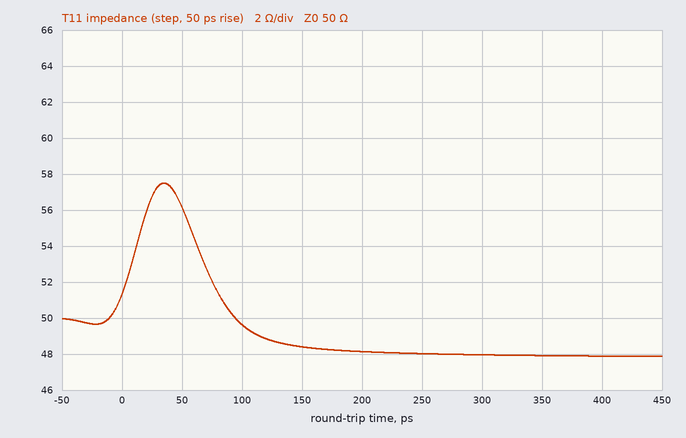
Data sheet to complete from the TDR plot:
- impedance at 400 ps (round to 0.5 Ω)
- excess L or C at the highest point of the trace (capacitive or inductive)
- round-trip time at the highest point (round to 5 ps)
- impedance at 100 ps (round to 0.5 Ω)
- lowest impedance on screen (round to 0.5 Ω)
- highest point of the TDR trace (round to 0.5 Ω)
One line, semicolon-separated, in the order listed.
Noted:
48.0 Ω; inductive; 35 ps; 49.5 Ω; 48.0 Ω; 57.5 Ω
